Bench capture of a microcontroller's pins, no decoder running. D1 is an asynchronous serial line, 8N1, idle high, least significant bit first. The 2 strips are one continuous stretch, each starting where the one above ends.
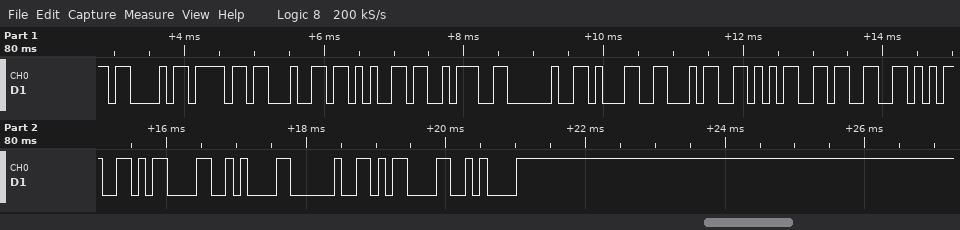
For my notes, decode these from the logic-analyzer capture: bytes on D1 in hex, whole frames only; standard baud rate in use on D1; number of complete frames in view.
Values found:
43 6F 64 65 3A 20 31 34 35 33 35 0D 0A 20 0D 0A
9600 baud
16
